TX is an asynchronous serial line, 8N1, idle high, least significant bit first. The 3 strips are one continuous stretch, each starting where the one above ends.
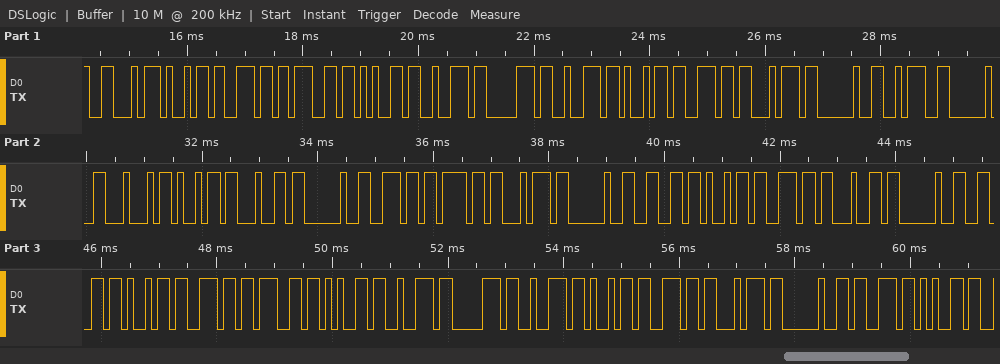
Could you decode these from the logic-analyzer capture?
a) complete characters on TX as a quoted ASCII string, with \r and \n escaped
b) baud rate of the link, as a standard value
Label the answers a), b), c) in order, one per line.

a) "Fingerprint : Did not find fingerprint se"
b) 9600 baud
